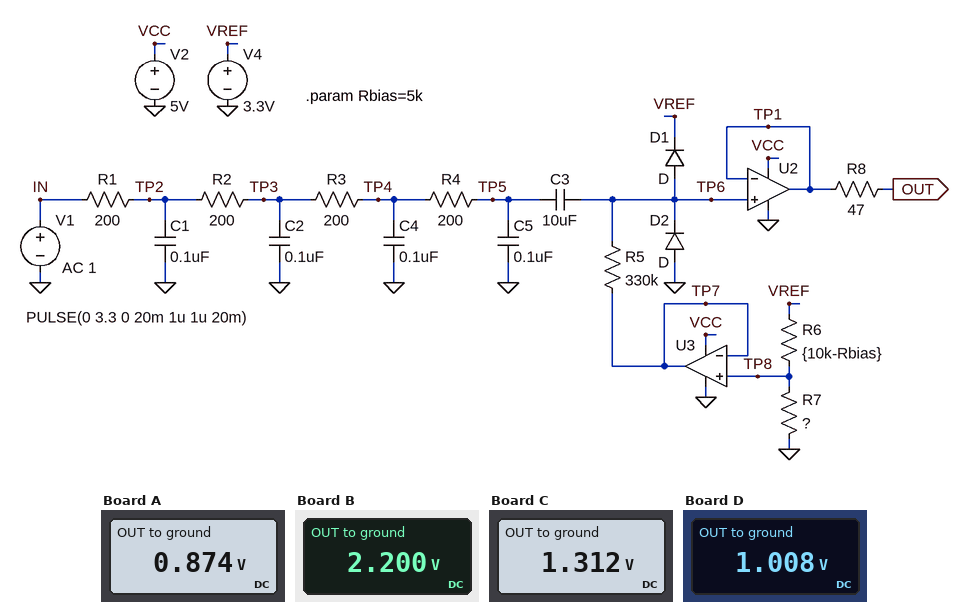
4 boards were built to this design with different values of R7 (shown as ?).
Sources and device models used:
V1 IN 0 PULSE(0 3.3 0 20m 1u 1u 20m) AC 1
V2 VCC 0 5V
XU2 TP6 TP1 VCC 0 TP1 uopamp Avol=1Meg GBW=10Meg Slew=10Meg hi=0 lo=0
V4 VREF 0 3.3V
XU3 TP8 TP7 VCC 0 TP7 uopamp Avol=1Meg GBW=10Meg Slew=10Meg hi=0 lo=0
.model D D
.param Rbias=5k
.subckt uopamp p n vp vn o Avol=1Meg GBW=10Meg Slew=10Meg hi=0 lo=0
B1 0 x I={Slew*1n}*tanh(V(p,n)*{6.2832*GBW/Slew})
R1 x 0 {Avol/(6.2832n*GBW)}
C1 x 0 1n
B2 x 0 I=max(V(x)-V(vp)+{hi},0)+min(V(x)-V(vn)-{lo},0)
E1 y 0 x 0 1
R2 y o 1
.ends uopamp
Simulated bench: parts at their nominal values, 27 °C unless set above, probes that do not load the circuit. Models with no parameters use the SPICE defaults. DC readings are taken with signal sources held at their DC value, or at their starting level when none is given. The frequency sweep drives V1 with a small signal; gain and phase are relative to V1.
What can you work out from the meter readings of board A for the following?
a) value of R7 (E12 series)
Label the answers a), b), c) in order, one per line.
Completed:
a) 1.8 kΩ
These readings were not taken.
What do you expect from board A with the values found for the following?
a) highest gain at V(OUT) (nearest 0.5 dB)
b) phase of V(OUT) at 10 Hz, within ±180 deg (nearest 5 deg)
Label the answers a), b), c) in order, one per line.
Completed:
a) 0 dB
b) 0 deg
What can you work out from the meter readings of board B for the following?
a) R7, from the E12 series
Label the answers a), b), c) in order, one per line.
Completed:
a) 10 kΩ
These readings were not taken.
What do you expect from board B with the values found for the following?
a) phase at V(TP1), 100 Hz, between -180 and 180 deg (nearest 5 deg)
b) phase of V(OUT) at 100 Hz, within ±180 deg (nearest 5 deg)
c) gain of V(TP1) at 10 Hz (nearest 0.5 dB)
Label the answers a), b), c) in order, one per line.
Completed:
a) -5 deg
b) -5 deg
c) 0 dB
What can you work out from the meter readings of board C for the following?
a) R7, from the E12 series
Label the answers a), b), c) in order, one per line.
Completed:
a) 3.3 kΩ
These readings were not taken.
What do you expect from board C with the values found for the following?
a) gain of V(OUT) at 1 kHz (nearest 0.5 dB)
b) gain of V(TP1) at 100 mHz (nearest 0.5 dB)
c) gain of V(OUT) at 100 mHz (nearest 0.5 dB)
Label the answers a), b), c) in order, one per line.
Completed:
a) -3.5 dB
b) -1.0 dB
c) -1.0 dB
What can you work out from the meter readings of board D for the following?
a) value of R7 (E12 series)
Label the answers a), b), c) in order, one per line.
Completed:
a) 2.2 kΩ
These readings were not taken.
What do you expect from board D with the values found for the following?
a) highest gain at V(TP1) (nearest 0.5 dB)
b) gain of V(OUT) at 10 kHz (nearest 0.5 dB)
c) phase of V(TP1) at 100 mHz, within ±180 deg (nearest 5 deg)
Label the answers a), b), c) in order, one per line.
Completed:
a) 0 dB
b) -26.0 dB
c) 25 deg
